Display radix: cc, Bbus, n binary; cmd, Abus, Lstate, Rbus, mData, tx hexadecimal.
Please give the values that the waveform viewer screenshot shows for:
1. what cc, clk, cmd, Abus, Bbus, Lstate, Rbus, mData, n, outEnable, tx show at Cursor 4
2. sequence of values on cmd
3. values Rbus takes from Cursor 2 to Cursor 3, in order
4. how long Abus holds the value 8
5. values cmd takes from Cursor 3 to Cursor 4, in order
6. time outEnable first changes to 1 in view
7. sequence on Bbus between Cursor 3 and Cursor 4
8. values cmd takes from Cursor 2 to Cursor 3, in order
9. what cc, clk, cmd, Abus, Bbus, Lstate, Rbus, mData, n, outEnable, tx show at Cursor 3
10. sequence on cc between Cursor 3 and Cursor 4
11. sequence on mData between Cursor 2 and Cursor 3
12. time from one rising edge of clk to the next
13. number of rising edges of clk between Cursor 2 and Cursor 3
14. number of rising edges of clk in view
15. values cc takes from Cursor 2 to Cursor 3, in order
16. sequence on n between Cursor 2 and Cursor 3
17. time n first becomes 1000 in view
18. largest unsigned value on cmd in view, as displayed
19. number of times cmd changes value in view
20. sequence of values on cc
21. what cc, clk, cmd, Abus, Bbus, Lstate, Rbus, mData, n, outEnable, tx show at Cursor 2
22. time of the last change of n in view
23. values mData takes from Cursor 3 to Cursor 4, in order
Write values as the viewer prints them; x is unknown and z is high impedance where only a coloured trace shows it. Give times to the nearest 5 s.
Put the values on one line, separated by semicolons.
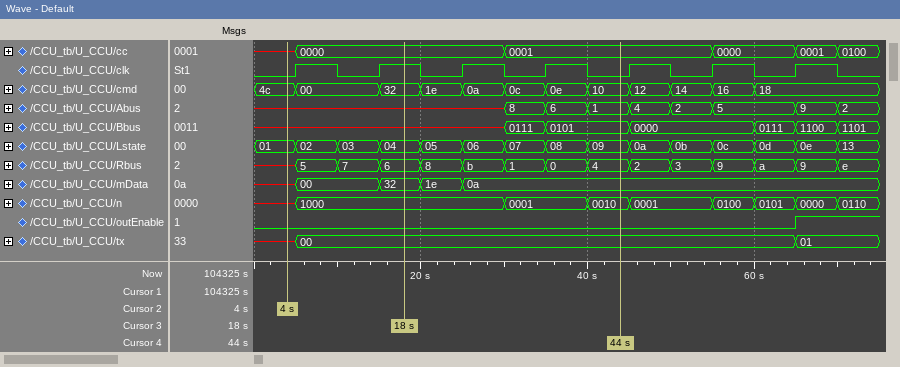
cc=0001, clk=0, cmd=10, Abus=1, Bbus=0101, Lstate=09, Rbus=4, mData=0a, n=0010, outEnable=0, tx=00; 4c, 00, 32, 1e, 0a, 0c, 0e, 10, 12, 14, 16, 18; x, 5, 7, 6; 5 s; 32, 1e, 0a, 0c, 0e, 10; 65 s; x, 0111, 0101; 4c, 00, 32; cc=0000, clk=1, cmd=32, Abus=x, Bbus=x, Lstate=04, Rbus=6, mData=32, n=1000, outEnable=0, tx=00; 0000, 0001; x, 00, 32; 10 s; 2; 7; x, 0000; x, 1000; 5 s; 4c; 11; x, 0000, 0001, 0000, 0001, 0100; cc=x, clk=0, cmd=4c, Abus=x, Bbus=x, Lstate=01, Rbus=x, mData=x, n=x, outEnable=0, tx=x; 70 s; 32, 1e, 0a
